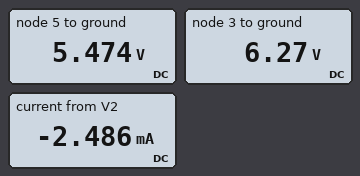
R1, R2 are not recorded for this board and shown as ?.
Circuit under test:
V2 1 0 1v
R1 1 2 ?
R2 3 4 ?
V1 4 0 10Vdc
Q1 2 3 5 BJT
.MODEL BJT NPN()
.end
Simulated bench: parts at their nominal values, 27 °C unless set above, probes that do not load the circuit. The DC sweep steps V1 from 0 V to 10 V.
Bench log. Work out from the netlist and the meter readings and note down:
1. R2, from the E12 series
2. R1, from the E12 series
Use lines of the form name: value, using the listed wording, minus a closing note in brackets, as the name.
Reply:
R2, from the E12 series: 1.5 kΩ
R1, from the E12 series: 1.8 kΩ
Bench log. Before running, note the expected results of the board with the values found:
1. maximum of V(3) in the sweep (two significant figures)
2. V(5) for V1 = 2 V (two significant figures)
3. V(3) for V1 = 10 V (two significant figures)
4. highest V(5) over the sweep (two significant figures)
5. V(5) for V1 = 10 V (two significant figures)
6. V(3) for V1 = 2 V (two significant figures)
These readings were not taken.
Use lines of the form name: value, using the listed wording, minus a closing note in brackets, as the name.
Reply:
maximum of V(3) in the sweep: 6.3 V
V(5) for V1 = 2 V: 1.2 V
V(3) for V1 = 10 V: 6.3 V
highest V(5) over the sweep: 5.5 V
V(5) for V1 = 10 V: 5.5 V
V(3) for V1 = 2 V: 1.9 V
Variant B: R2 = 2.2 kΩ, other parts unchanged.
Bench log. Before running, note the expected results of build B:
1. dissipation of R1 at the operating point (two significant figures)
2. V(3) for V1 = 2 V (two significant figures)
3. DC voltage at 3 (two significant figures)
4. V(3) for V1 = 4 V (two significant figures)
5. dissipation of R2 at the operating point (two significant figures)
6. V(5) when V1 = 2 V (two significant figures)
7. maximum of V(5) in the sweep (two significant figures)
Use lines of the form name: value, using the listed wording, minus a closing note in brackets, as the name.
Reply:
dissipation of R1 at the operating point: 7.6 mW
V(3) for V1 = 2 V: 1.8 V
DC voltage at 3: 5.5 V
V(3) for V1 = 4 V: 2.8 V
dissipation of R2 at the operating point: 9.3 mW
V(5) when V1 = 2 V: 1.1 V
maximum of V(5) in the sweep: 4.7 V
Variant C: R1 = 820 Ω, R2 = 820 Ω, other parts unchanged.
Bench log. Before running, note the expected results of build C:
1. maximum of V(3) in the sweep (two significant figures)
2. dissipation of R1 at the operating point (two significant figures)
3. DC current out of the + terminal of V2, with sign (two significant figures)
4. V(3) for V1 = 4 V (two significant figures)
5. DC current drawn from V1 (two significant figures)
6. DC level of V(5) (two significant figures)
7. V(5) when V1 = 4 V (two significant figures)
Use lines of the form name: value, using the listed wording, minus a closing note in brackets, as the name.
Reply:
maximum of V(3) in the sweep: 5.9 V
dissipation of R1 at the operating point: 20 mW
DC current out of the + terminal of V2, with sign: -5.0 mA
V(3) for V1 = 4 V: 2.9 V
DC current drawn from V1: 5.0 mA
DC level of V(5): 5.1 V
V(5) when V1 = 4 V: 2.1 V
